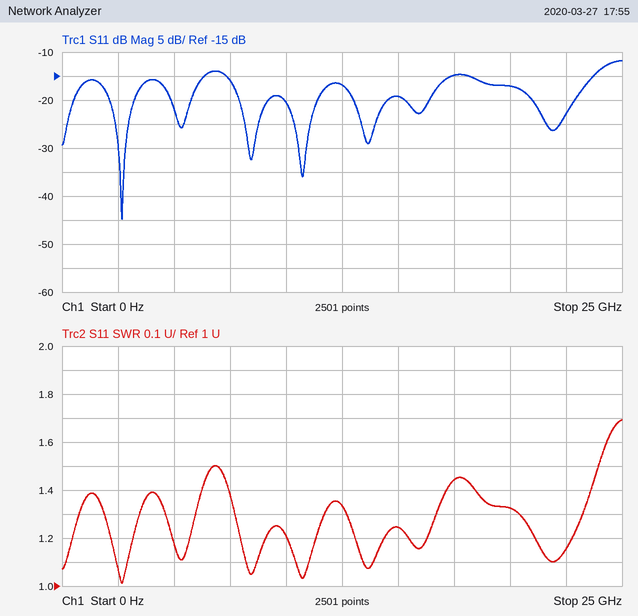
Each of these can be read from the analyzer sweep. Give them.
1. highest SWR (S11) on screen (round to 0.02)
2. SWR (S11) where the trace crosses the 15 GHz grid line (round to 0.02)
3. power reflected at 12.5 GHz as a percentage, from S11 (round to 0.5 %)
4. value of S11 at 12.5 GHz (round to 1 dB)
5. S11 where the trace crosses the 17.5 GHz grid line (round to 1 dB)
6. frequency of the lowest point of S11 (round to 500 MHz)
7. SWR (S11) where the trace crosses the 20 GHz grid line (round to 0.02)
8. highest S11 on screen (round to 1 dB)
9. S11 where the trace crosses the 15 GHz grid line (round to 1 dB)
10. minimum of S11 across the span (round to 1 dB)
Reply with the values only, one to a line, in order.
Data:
1.70
1.24
2.0 %
-17 dB
-15 dB
2.5 GHz
1.32
-12 dB
-19 dB
-45 dB
